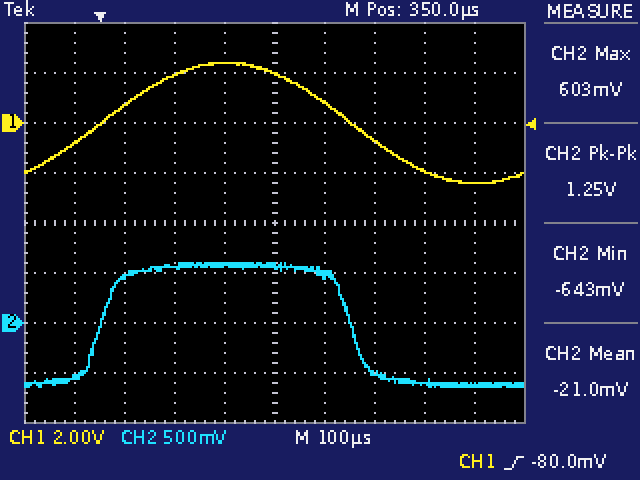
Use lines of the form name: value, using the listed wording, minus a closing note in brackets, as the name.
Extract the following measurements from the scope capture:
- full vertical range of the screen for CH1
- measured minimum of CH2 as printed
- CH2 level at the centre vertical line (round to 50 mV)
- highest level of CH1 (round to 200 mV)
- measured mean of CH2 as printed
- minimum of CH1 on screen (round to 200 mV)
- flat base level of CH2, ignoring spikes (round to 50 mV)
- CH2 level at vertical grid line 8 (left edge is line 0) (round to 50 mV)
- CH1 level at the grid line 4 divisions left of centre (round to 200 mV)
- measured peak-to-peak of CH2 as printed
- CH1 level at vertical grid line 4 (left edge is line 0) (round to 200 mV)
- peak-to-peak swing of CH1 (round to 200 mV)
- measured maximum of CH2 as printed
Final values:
full vertical range of the screen for CH1: 16 V
measured minimum of CH2 as printed: -643 mV
CH2 level at the centre vertical line: 550 mV
highest level of CH1: 2.4 V
measured mean of CH2 as printed: -21.0 mV
minimum of CH1 on screen: -2.4 V
flat base level of CH2, ignoring spikes: -600 mV
CH2 level at vertical grid line 8 (left edge is line 0): -600 mV
CH1 level at the grid line 4 divisions left of centre: -800 mV
measured peak-to-peak of CH2 as printed: 1.25 V
CH1 level at vertical grid line 4 (left edge is line 0): 2.4 V
peak-to-peak swing of CH1: 4.8 V
measured maximum of CH2 as printed: 603 mV
